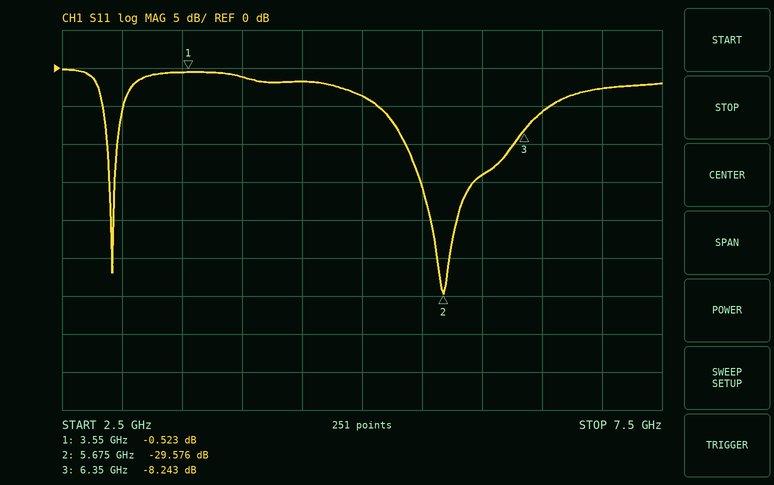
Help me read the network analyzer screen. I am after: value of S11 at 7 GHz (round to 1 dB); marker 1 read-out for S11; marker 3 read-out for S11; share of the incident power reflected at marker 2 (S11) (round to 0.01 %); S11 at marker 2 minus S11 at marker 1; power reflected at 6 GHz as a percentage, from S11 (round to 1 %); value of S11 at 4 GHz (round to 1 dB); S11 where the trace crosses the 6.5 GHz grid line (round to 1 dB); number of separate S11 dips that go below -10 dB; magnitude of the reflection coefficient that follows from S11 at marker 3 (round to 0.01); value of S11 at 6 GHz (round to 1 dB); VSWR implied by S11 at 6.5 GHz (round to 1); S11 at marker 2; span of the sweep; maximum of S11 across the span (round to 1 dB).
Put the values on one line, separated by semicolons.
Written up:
-3 dB; -0.523 dB; -8.243 dB; 0.11 %; -29.053 dB; 4 %; -1 dB; -6 dB; 2; 0.39; -14 dB; 3; -29.576 dB; 5 GHz; 0 dB
